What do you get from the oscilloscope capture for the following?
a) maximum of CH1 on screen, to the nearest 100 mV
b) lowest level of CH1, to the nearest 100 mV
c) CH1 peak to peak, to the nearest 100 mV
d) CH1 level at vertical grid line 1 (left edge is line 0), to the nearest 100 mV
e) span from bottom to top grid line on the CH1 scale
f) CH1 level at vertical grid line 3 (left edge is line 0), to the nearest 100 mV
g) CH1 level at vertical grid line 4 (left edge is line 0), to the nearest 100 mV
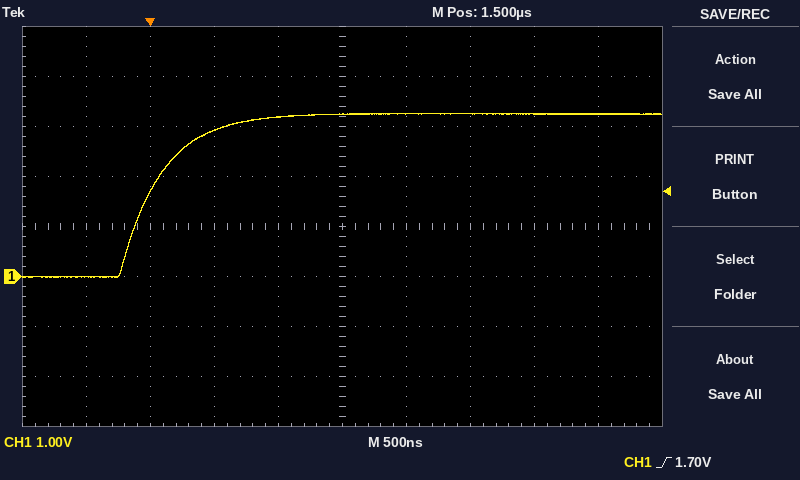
3.3 V
0.0 V
3.3 V
0.0 V
8 V
2.9 V
3.2 V
